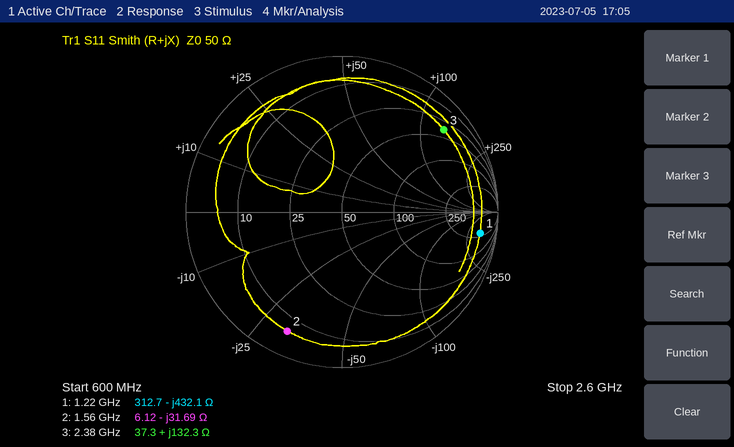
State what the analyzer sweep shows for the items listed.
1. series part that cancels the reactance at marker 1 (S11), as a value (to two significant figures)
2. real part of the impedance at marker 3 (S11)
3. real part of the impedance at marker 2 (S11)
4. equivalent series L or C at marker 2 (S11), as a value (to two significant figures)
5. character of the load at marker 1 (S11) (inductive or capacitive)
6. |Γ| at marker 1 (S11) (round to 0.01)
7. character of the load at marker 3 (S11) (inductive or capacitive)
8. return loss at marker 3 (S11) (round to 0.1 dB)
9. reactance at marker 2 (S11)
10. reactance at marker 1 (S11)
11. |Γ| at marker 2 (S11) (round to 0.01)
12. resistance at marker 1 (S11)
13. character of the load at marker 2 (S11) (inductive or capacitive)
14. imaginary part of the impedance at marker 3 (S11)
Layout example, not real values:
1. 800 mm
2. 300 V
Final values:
1. 56 nH
2. 37.3 Ω
3. 6.12 Ω
4. 3.2 pF
5. capacitive
6. 0.90
7. inductive
8. 1.5 dB
9. -31.69 Ω
10. -432.1 Ω
11. 0.84
12. 312.7 Ω
13. capacitive
14. +132.3 Ω
